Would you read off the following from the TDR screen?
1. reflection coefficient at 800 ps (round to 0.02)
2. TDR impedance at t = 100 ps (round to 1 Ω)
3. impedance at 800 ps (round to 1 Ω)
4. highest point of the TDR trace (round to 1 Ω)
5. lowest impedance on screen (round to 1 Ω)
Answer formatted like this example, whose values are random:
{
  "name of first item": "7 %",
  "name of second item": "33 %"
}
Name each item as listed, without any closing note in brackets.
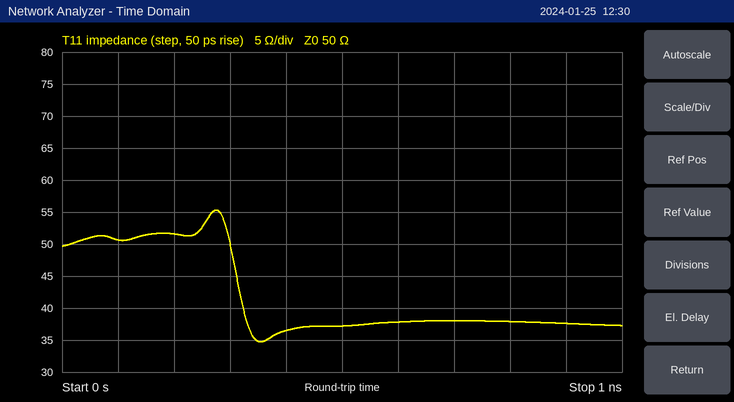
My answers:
{
  "reflection coefficient at 800 ps": "-0.14",
  "TDR impedance at t = 100 ps": "51 Ω",
  "impedance at 800 ps": "38 Ω",
  "highest point of the TDR trace": "55 Ω",
  "lowest impedance on screen": "35 Ω"
}
